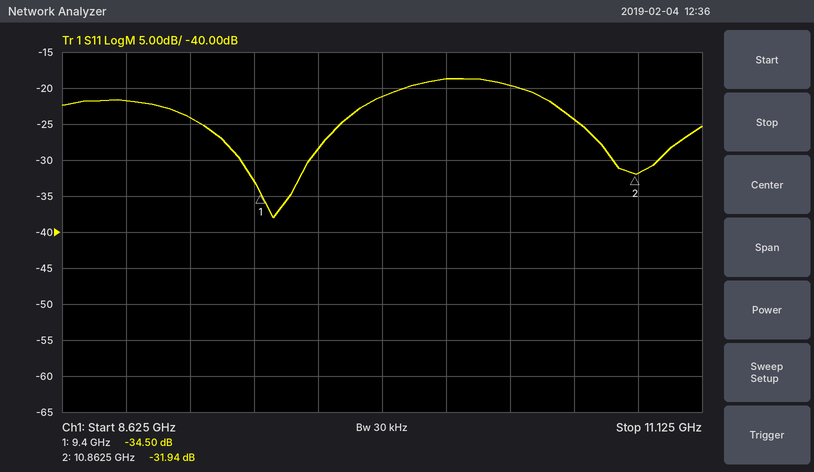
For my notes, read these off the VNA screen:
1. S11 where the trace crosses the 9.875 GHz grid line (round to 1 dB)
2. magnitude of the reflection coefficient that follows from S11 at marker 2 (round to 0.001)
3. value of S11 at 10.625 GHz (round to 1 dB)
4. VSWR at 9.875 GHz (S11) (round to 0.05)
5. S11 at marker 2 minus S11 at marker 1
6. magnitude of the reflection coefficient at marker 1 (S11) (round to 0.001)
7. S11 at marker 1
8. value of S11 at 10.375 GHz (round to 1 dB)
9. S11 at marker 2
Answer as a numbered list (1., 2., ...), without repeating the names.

1. -21 dB
2. 0.025
3. -24 dB
4. 1.20
5. 2.56 dB
6. 0.019
7. -34.50 dB
8. -20 dB
9. -31.94 dB
